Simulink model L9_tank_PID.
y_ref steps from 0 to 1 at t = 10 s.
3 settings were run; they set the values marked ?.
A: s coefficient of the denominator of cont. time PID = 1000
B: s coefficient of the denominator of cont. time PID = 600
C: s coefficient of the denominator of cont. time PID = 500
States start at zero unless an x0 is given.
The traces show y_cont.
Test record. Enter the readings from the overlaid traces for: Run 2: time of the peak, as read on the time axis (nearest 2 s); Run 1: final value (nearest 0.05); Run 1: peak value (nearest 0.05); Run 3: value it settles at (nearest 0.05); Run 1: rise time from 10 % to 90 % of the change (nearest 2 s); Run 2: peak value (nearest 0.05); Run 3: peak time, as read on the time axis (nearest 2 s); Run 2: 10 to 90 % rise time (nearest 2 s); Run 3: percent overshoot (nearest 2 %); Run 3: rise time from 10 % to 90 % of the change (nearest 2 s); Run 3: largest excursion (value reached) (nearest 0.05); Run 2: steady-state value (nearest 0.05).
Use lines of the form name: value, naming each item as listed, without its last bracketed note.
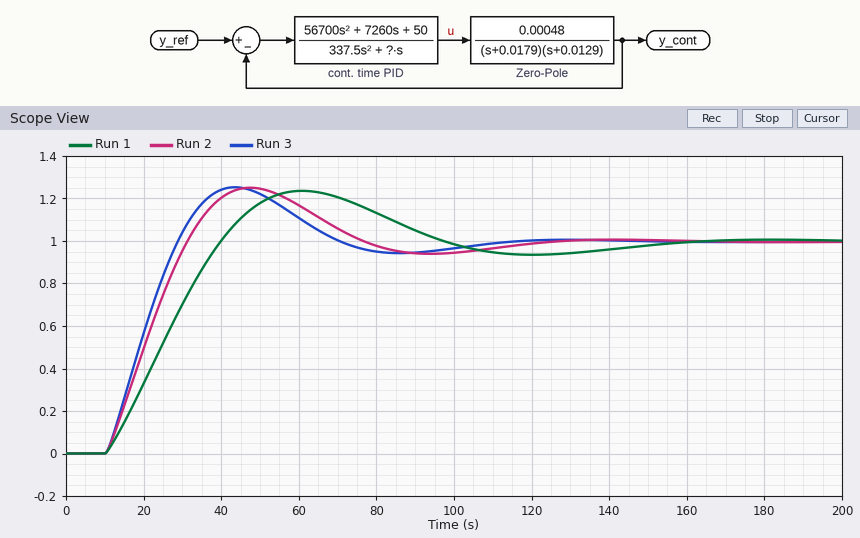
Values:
Run 2: time of the peak, as read on the time axis: 48 s
Run 1: final value: 1.00
Run 1: peak value: 1.25
Run 3: value it settles at: 1.00
Run 1: rise time from 10 % to 90 % of the change: 22 s
Run 2: peak value: 1.25
Run 3: peak time, as read on the time axis: 44 s
Run 2: 10 to 90 % rise time: 16 s
Run 3: percent overshoot: 26 %
Run 3: rise time from 10 % to 90 % of the change: 14 s
Run 3: largest excursion (value reached): 1.25
Run 2: steady-state value: 1.00
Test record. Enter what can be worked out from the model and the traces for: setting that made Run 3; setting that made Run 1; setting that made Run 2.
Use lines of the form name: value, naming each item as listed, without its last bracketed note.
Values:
setting that made Run 3: C
setting that made Run 1: A
setting that made Run 2: B
